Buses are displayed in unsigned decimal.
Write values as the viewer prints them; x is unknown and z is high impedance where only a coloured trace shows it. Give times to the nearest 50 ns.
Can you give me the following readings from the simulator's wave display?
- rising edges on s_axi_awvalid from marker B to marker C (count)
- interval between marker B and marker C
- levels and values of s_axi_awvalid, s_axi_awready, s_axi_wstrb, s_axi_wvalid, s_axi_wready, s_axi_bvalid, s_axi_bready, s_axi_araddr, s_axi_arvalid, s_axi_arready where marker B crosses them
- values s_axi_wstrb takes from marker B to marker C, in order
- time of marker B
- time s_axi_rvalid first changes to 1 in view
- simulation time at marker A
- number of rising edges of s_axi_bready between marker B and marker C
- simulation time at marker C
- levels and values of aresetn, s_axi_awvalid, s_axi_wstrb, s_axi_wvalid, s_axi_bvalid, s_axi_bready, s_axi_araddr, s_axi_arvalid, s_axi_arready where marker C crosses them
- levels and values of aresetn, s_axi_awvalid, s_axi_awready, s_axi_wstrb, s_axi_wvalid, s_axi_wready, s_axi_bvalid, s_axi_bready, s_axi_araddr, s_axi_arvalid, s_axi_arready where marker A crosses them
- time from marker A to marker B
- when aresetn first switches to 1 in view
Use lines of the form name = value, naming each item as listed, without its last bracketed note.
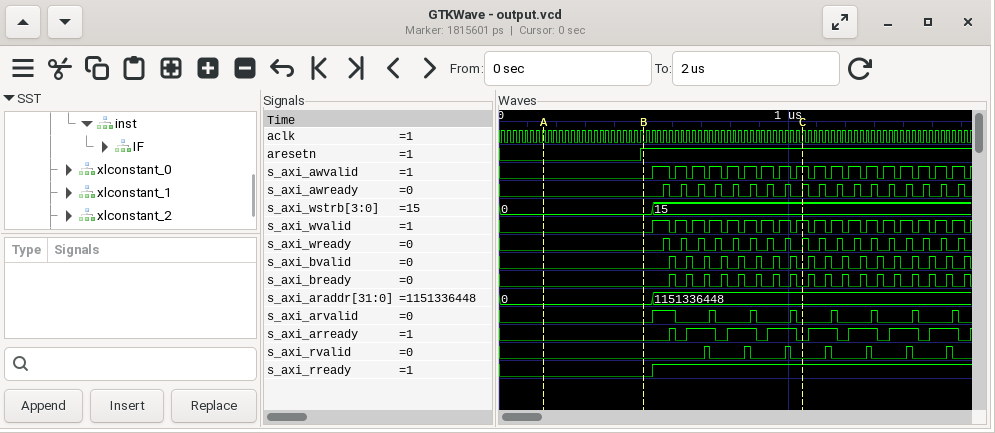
rising edges on s_axi_awvalid from marker B to marker C = 9
interval between marker B and marker C = 550 ns
levels and values of s_axi_awvalid, s_axi_awready, s_axi_wstrb, s_axi_wvalid, s_axi_wready, s_axi_bvalid, s_axi_bready, s_axi_araddr, s_axi_arvalid, s_axi_arready where marker B crosses them = s_axi_awvalid=0, s_axi_awready=0, s_axi_wstrb=0, s_axi_wvalid=0, s_axi_wready=0, s_axi_bvalid=0, s_axi_bready=0, s_axi_araddr=0, s_axi_arvalid=0, s_axi_arready=0
values s_axi_wstrb takes from marker B to marker C, in order = 0, 15
time of marker B = 500 ns
time s_axi_rvalid first changes to 1 in view = 700 ns
simulation time at marker A = 150 ns
number of rising edges of s_axi_bready between marker B and marker C = 8
simulation time at marker C = 1050 ns
levels and values of aresetn, s_axi_awvalid, s_axi_wstrb, s_axi_wvalid, s_axi_bvalid, s_axi_bready, s_axi_araddr, s_axi_arvalid, s_axi_arready where marker C crosses them = aresetn=1, s_axi_awvalid=1, s_axi_wstrb=15, s_axi_wvalid=1, s_axi_bvalid=0, s_axi_bready=0, s_axi_araddr=1151336448, s_axi_arvalid=0, s_axi_arready=0
levels and values of aresetn, s_axi_awvalid, s_axi_awready, s_axi_wstrb, s_axi_wvalid, s_axi_wready, s_axi_bvalid, s_axi_bready, s_axi_araddr, s_axi_arvalid, s_axi_arready where marker A crosses them = aresetn=0, s_axi_awvalid=0, s_axi_awready=0, s_axi_wstrb=0, s_axi_wvalid=0, s_axi_wready=0, s_axi_bvalid=0, s_axi_bready=0, s_axi_araddr=0, s_axi_arvalid=0, s_axi_arready=0
time from marker A to marker B = 350 ns
when aresetn first switches to 1 in view = 500 ns
